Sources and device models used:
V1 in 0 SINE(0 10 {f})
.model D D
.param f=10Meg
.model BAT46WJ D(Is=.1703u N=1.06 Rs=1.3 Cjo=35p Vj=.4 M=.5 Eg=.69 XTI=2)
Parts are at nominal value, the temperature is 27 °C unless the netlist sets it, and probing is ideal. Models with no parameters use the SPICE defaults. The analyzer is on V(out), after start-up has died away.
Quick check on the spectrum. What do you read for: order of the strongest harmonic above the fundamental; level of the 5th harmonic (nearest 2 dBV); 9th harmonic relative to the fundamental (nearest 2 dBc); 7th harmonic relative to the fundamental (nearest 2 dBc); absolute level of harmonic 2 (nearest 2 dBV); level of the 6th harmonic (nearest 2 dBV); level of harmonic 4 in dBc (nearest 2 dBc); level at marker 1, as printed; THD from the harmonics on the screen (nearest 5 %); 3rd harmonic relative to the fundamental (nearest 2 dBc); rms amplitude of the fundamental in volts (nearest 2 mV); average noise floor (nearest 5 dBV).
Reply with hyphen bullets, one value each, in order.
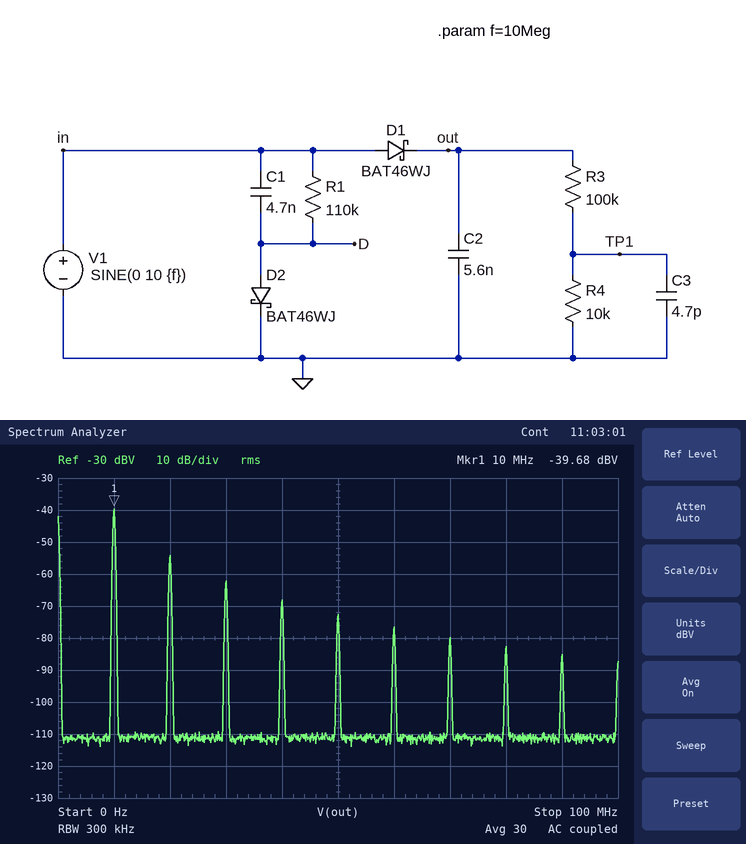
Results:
- 2
- -72 dBV
- -46 dBc
- -40 dBc
- -54 dBV
- -76 dBV
- -28 dBc
- -39.68 dBV
- 20 %
- -22 dBc
- 10 mV
- -110 dBV
